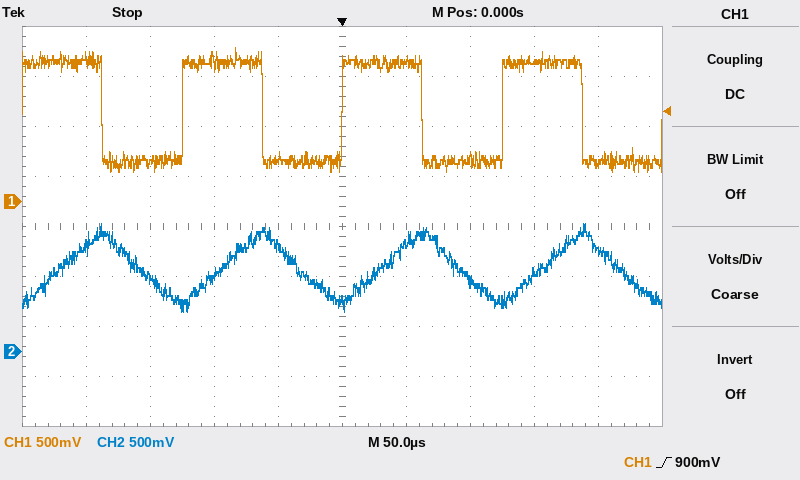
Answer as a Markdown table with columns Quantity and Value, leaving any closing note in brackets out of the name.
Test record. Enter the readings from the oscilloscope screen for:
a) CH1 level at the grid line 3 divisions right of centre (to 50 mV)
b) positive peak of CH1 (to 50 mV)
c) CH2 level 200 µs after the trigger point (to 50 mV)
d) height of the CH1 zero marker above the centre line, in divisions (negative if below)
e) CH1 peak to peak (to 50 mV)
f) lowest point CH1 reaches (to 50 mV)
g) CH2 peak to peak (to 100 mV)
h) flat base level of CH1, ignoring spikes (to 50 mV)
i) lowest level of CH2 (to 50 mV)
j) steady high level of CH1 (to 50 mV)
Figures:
| Quantity | Value |
|---|---|
| CH1 level at the grid line 3 divisions right of centre | 1.40 V |
| positive peak of CH1 | 1.55 V |
| CH2 level 200 µs after the trigger point | 1.00 V |
| height of the CH1 zero marker above the centre line, in divisions | +0.5 div |
| CH1 peak to peak | 1.25 V |
| lowest point CH1 reaches | 300 mV |
| CH2 peak to peak | 900 mV |
| flat base level of CH1, ignoring spikes | 400 mV |
| lowest level of CH2 | 400 mV |
| steady high level of CH1 | 1.40 V |
